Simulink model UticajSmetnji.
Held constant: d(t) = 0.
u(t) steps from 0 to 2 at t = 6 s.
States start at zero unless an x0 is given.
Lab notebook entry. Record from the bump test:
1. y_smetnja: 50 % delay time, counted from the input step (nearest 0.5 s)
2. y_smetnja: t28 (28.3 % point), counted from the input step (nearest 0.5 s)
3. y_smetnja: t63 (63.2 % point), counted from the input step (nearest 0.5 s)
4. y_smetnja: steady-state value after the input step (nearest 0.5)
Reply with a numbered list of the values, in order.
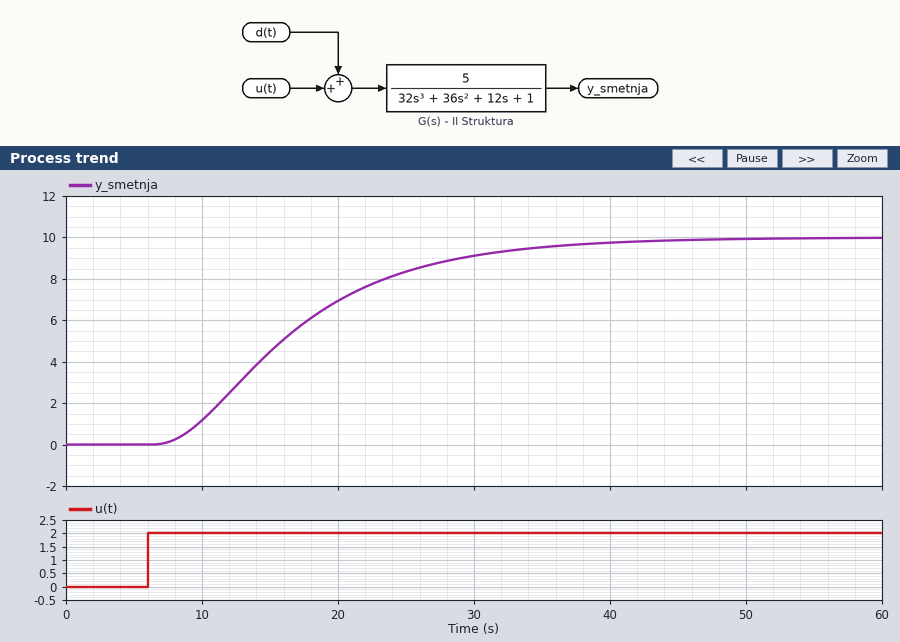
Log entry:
1. 10.0 s
2. 6.5 s
3. 12.5 s
4. 10.0
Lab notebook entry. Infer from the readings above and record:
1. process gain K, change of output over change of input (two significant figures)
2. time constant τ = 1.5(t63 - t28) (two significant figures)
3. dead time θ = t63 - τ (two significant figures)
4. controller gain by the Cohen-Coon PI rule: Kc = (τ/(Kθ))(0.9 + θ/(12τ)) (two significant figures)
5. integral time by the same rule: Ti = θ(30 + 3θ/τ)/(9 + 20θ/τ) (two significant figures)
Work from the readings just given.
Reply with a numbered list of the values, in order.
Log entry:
1. 5.0
2. 9.0 s
3. 3.5 s
4. 0.48
5. 6.5 s
